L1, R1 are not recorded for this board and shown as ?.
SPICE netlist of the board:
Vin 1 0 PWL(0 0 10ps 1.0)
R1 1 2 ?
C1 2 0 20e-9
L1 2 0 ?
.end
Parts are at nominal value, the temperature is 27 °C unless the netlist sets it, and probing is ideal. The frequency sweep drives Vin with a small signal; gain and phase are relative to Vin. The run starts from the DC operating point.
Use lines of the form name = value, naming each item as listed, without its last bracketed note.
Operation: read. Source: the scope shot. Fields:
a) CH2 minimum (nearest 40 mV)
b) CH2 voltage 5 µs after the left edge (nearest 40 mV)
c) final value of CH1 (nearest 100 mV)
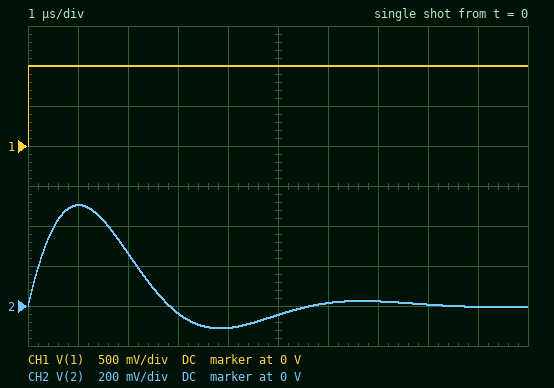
CH2 minimum = -120 mV
CH2 voltage 5 µs after the left edge = -40 mV
final value of CH1 = 1.0 V
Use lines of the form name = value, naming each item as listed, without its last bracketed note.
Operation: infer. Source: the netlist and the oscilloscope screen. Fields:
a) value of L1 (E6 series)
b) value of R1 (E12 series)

value of L1 = 33 µH
value of R1 = 47 Ω
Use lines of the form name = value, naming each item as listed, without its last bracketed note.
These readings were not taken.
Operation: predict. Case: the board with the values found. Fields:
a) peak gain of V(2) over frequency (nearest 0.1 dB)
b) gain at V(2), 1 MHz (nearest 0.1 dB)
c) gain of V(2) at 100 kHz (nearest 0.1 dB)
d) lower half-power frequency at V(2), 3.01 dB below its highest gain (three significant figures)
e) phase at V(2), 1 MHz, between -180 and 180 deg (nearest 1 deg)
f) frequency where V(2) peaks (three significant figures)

peak gain of V(2) over frequency = 0 dB
gain at V(2), 1 MHz = -15.2 dB
gain of V(2) at 100 kHz = -5.8 dB
lower half-power frequency at V(2), 3.01 dB below its highest gain = 129 kHz
phase at V(2), 1 MHz, between -180 and 180 deg = -80 deg
frequency where V(2) peaks = 196 kHz
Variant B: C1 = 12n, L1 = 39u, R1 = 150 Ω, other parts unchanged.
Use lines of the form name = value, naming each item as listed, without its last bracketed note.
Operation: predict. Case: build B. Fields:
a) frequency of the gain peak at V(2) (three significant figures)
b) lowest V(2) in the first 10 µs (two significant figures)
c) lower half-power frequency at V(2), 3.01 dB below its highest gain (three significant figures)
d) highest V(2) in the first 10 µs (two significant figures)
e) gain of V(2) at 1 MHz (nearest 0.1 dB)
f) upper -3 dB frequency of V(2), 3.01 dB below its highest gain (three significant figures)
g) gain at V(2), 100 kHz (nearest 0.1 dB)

frequency of the gain peak at V(2) = 233 kHz
lowest V(2) in the first 10 µs = -160 mV
lower half-power frequency at V(2), 3.01 dB below its highest gain = 193 kHz
highest V(2) in the first 10 µs = 290 mV
gain of V(2) at 1 MHz = -20.6 dB
upper -3 dB frequency of V(2), 3.01 dB below its highest gain = 281 kHz
gain at V(2), 100 kHz = -14.1 dB
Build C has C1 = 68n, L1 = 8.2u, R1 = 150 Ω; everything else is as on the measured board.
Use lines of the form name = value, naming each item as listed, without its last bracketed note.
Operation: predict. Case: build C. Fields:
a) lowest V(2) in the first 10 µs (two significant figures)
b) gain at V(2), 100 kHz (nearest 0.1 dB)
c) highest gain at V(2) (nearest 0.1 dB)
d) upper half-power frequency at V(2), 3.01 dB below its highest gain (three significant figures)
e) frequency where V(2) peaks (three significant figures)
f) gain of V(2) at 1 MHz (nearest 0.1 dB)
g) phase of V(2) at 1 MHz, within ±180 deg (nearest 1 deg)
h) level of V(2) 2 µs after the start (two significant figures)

lowest V(2) in the first 10 µs = -62 mV
gain at V(2), 100 kHz = -27.1 dB
highest gain at V(2) = 0 dB
upper half-power frequency at V(2), 3.01 dB below its highest gain = 221 kHz
frequency where V(2) peaks = 213 kHz
gain of V(2) at 1 MHz = -35.7 dB
phase of V(2) at 1 MHz, within ±180 deg = -89 deg
level of V(2) 2 µs after the start = 30 mV
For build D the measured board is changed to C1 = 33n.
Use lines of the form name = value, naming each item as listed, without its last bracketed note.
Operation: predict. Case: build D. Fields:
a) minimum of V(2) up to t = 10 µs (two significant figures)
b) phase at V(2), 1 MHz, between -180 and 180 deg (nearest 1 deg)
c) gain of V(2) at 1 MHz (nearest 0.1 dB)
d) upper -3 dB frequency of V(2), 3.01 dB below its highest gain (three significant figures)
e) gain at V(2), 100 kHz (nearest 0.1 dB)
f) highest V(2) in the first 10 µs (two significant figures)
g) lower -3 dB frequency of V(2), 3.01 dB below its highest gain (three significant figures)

minimum of V(2) up to t = 10 µs = -140 mV
phase at V(2), 1 MHz, between -180 and 180 deg = -84 deg
gain of V(2) at 1 MHz = -19.6 dB
upper -3 dB frequency of V(2), 3.01 dB below its highest gain = 212 kHz
gain at V(2), 100 kHz = -4.3 dB
highest V(2) in the first 10 µs = 430 mV
lower -3 dB frequency of V(2), 3.01 dB below its highest gain = 110 kHz
